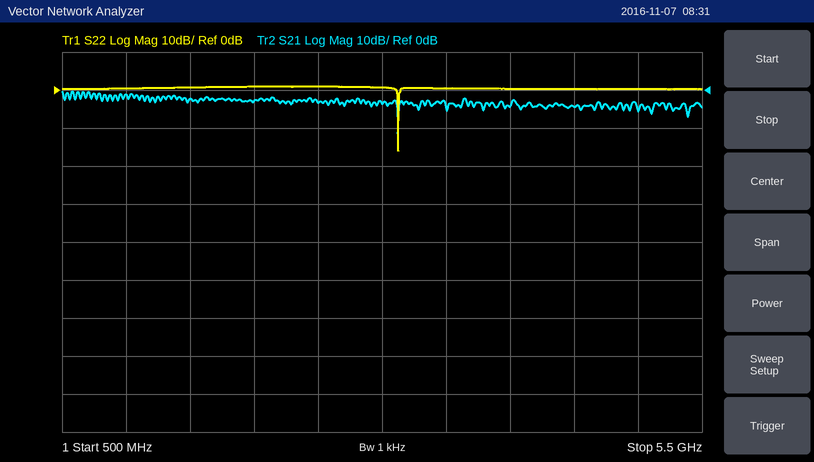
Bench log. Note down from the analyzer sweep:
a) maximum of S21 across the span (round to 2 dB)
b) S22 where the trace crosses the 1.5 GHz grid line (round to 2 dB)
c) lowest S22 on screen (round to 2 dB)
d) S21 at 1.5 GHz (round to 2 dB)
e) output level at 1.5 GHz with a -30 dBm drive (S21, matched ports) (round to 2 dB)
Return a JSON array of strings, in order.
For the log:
["0 dB", "0 dB", "-16 dB", "-2 dB", "-32 dBm"]
